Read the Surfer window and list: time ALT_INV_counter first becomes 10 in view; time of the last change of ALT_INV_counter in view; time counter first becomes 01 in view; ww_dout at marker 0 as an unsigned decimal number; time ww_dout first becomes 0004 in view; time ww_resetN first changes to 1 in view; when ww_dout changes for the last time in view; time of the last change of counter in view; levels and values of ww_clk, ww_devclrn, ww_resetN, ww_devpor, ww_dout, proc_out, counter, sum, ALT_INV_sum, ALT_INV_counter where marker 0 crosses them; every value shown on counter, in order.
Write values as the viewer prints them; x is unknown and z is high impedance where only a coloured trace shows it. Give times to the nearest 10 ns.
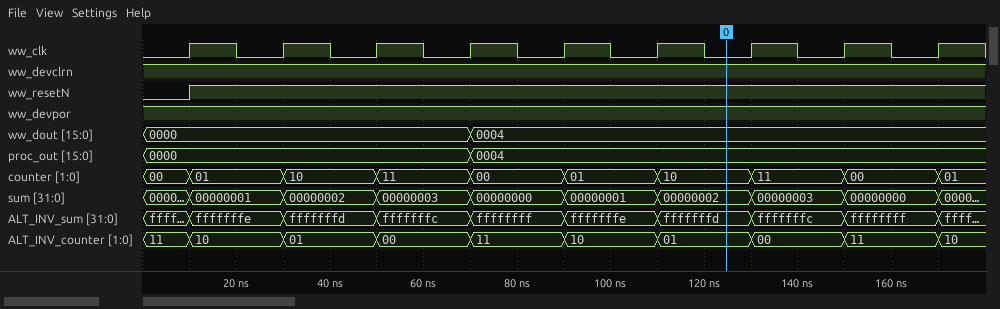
10 ns
170 ns
10 ns
4
70 ns
10 ns
70 ns
170 ns
ww_clk=0, ww_devclrn=1, ww_resetN=1, ww_devpor=1, ww_dout=0004, proc_out=0004, counter=10, sum=00000002, ALT_INV_sum=fffffffd, ALT_INV_counter=01
00, 01, 10, 11, 00, 01, 10, 11, 00, 01
